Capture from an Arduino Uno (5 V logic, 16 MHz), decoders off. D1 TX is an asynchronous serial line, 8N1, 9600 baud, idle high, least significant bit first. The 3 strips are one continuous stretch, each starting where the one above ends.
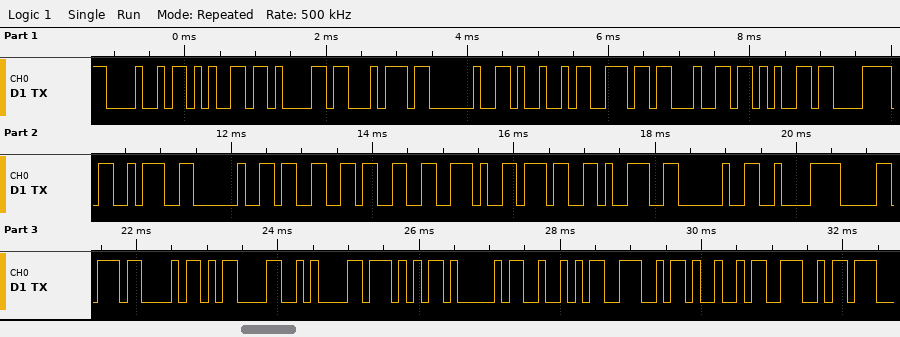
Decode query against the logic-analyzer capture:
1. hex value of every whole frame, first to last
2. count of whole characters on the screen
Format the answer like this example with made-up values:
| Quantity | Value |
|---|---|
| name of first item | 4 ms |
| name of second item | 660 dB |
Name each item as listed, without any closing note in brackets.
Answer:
| Quantity | Value |
|---|---|
| hex value of every whole frame, first to last | 48 65 61 74 20 49 6E 64 65 78 3A 20 33 33 2E 37 39 20 C2 B0 43 0D 0A 57 41 52 4E 49 4E |
| count of whole characters on the screen | 29 |
